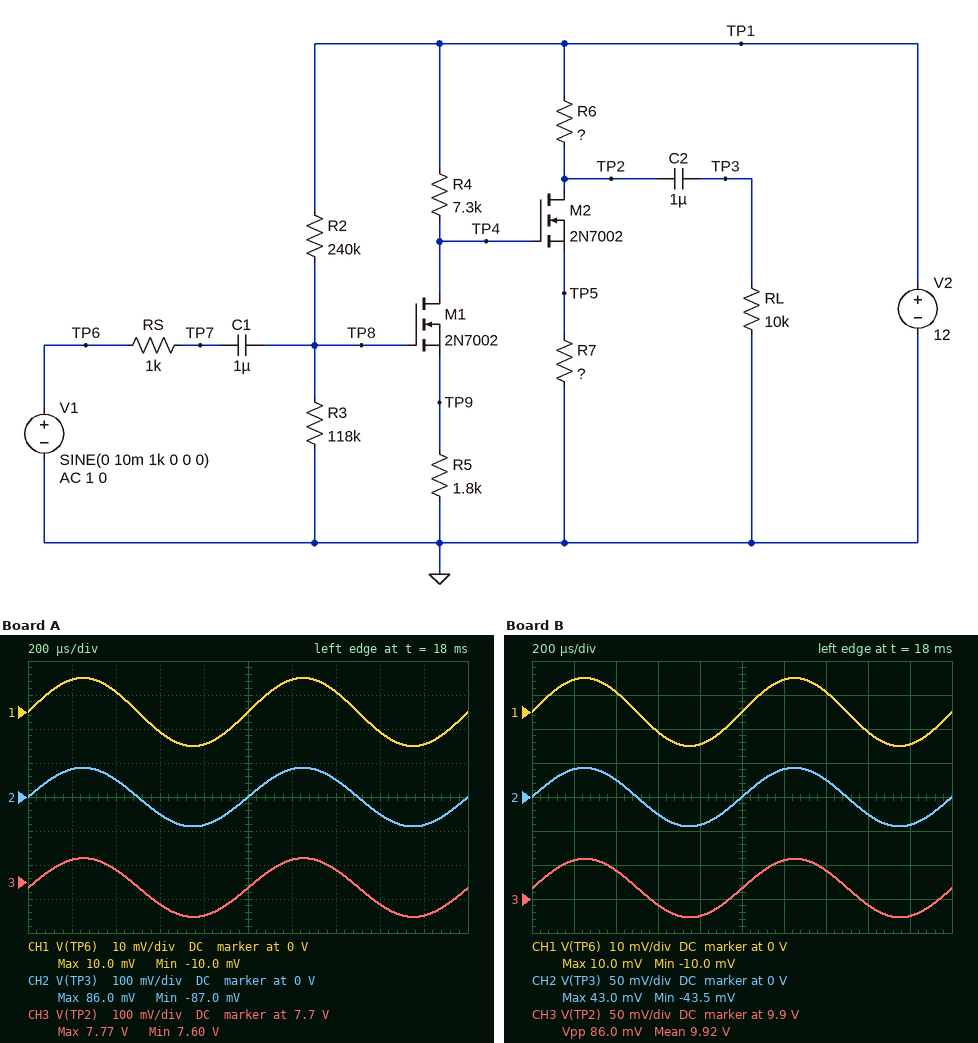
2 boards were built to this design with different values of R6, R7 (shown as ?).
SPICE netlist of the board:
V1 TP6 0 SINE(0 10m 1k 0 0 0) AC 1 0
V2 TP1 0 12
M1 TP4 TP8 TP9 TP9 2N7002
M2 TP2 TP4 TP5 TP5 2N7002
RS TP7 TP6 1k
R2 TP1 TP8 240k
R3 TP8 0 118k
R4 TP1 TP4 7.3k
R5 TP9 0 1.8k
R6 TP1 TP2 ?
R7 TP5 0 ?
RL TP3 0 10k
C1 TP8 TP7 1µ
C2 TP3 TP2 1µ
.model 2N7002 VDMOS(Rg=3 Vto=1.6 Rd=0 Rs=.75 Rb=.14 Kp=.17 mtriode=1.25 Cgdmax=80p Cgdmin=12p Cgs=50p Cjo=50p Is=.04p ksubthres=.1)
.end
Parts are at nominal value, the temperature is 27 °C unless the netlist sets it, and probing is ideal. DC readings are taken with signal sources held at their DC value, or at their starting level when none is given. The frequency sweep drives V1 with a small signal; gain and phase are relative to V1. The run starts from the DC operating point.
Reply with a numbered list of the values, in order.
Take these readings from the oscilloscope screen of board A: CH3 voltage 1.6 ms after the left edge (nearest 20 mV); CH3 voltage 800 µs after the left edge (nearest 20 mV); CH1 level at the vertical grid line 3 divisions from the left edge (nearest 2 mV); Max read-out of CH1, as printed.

1. 7.64 V
2. 7.60 V
3. -6 mV
4. 10.0 mV
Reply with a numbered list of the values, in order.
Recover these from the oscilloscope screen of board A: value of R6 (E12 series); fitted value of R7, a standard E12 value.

1. 5.6 kΩ
2. 1.5 kΩ
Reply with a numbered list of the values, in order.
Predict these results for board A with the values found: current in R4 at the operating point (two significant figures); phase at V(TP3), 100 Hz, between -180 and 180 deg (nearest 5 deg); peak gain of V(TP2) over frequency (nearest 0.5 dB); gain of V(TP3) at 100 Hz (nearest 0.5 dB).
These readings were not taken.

1. 1.3 mA
2. 5 deg
3. 21.5 dB
4. 18.5 dB
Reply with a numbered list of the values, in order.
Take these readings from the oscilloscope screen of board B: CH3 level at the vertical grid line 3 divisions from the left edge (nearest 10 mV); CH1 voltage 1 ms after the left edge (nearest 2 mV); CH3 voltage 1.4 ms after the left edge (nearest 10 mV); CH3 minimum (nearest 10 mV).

1. 9.89 V
2. 0 V
3. 9.94 V
4. 9.87 V
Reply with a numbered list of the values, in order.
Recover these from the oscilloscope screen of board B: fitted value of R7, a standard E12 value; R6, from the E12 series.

1. 2.7 kΩ
2. 4.7 kΩ
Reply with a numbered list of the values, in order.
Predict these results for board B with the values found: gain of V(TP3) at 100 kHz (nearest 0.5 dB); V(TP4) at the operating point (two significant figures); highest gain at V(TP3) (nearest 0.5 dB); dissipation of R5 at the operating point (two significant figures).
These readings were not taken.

1. 11.0 dB
2. 2.8 V
3. 12.5 dB
4. 2.9 mW
